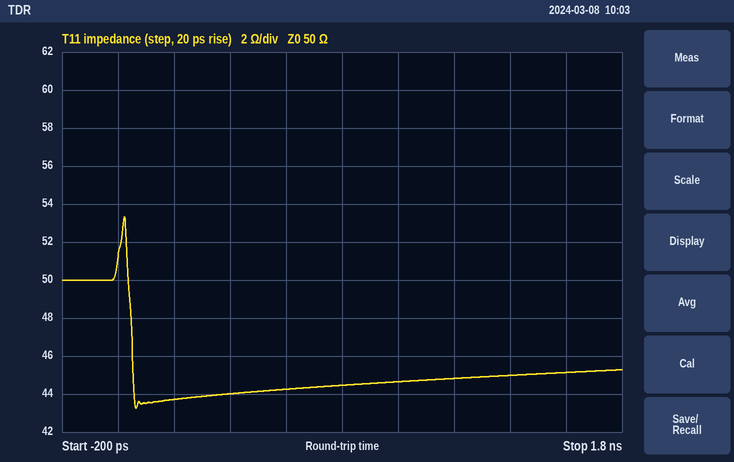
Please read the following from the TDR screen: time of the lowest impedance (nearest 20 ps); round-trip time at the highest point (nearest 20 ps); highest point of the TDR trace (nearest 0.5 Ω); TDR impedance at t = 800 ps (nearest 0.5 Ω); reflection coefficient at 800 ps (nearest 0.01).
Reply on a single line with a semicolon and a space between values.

60 ps; 20 ps; 53.5 Ω; 44.5 Ω; -0.06
